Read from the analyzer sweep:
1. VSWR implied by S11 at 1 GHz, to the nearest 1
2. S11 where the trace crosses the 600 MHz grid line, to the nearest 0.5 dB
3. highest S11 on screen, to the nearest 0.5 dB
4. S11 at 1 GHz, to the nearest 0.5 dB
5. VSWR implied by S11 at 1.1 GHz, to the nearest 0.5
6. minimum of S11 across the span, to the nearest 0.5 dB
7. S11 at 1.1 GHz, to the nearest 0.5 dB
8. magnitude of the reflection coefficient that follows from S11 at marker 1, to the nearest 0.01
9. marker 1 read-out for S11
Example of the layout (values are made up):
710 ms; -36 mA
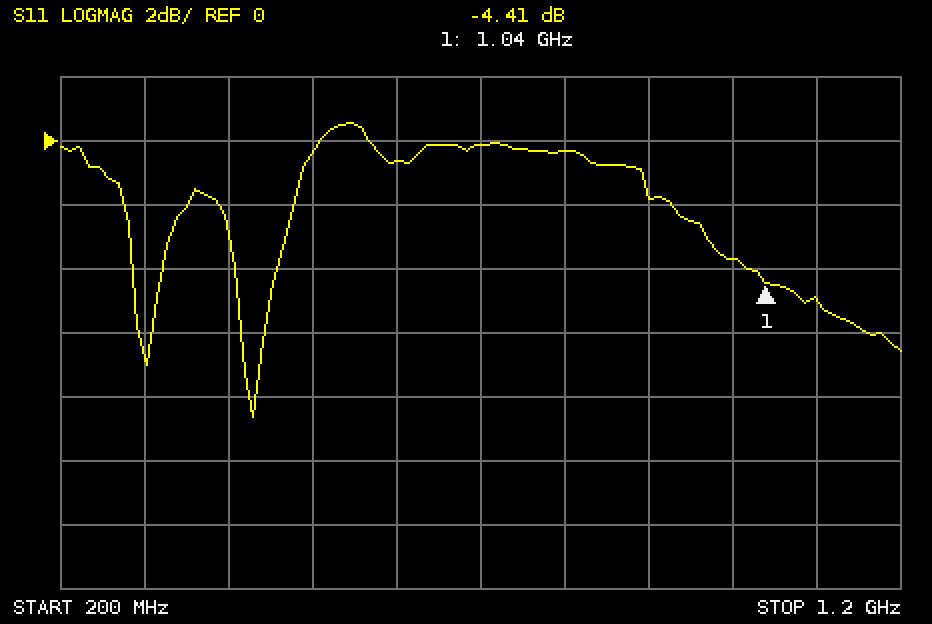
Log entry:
5; -0.5 dB; 0.5 dB; -3.5 dB; 3.5; -8.5 dB; -5.0 dB; 0.60; -4.41 dB
